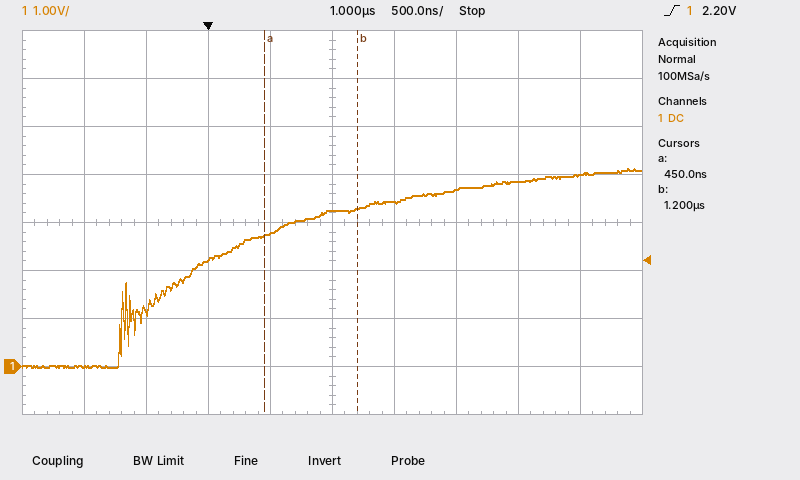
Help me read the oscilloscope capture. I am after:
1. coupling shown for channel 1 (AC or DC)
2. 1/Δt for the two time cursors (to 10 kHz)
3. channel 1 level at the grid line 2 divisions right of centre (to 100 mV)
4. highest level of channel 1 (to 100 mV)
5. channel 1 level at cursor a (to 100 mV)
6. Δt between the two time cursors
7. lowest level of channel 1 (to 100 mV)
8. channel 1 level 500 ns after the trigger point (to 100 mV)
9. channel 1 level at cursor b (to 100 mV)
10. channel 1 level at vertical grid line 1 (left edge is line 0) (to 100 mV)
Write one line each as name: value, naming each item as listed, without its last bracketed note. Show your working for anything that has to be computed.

coupling shown for channel 1: DC
1/Δt for the two time cursors: 1 / 750 ns ≈ 1.33 MHz
channel 1 level at the grid line 2 divisions right of centre: 3.7 V
highest level of channel 1: 4.1 V
channel 1 level at cursor a: 2.7 V
Δt between the two time cursors: 1.2 µs − (450 ns) = 750 ns
lowest level of channel 1: 0.0 V
channel 1 level 500 ns after the trigger point: 2.8 V
channel 1 level at cursor b: 3.3 V
channel 1 level at vertical grid line 1 (left edge is line 0): 0.0 V
